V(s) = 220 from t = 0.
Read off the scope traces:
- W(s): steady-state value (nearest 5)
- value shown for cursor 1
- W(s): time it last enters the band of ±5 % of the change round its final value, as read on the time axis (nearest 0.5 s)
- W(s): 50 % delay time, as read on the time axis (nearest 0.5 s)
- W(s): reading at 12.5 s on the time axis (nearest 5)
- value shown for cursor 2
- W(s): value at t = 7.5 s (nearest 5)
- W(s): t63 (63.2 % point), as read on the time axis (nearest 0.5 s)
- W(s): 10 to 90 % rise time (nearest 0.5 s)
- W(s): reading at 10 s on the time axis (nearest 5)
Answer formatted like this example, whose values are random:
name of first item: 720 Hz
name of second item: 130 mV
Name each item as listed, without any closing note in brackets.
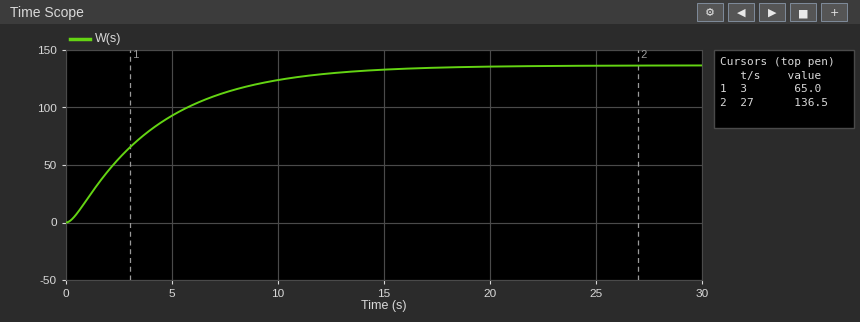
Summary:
W(s): steady-state value: 135
value shown for cursor 1: 65.0
W(s): time it last enters the band of ±5 % of the change round its final value, as read on the time axis: 12.5 s
W(s): 50 % delay time, as read on the time axis: 3.0 s
W(s): reading at 12.5 s on the time axis: 130
value shown for cursor 2: 136.5
W(s): value at t = 7.5 s: 115
W(s): t63 (63.2 % point), as read on the time axis: 4.5 s
W(s): 10 to 90 % rise time: 9.0 s
W(s): reading at 10 s on the time axis: 125
